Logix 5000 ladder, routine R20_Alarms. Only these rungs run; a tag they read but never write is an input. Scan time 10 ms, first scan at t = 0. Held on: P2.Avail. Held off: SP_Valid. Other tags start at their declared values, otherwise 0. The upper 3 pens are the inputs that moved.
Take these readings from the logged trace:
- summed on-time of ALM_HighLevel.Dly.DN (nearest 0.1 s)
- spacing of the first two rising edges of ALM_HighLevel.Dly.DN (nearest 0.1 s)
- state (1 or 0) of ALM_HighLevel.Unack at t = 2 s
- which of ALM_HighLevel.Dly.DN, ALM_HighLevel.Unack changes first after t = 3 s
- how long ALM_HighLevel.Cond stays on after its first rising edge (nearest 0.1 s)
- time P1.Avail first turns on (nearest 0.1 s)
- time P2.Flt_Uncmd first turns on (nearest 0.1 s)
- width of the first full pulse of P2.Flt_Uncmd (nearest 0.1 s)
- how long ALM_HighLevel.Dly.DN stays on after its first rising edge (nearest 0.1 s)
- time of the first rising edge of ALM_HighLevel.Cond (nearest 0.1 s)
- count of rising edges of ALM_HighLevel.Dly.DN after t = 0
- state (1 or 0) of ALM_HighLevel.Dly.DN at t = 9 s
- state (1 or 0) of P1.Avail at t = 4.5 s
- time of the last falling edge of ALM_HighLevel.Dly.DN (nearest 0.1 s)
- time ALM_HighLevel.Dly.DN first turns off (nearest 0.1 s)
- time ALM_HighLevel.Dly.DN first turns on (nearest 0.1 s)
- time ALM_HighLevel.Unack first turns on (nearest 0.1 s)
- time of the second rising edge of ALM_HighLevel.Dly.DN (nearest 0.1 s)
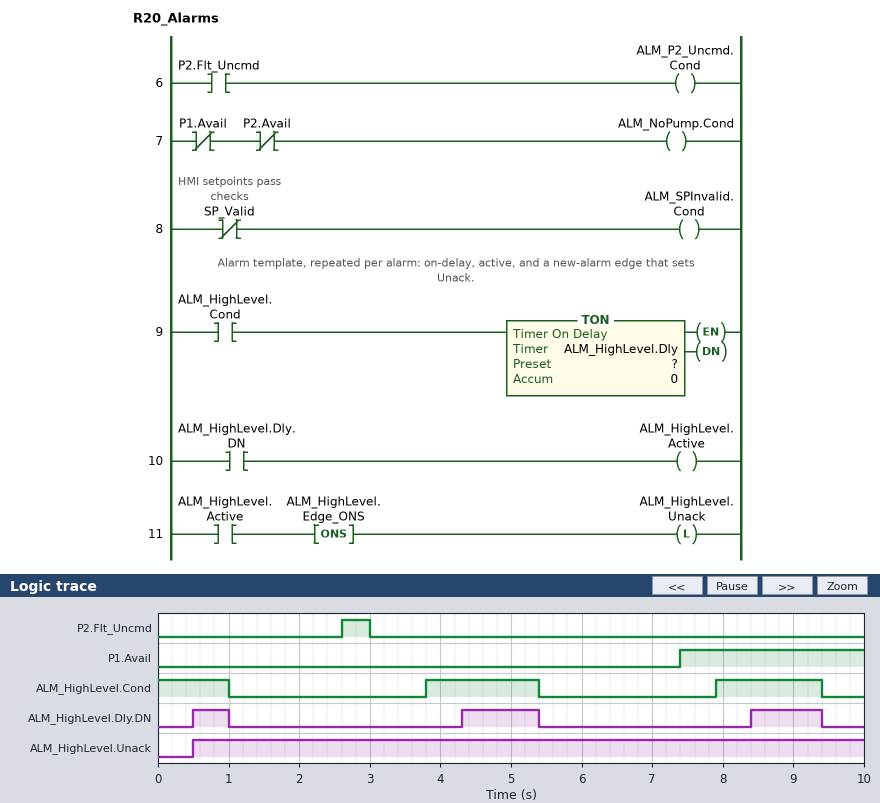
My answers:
2.6 s
3.8 s
1
ALM_HighLevel.Dly.DN
1.6 s
7.4 s
2.6 s
0.4 s
0.5 s
3.8 s
3
1
0
9.4 s
1.0 s
0.5 s
0.5 s
4.3 s
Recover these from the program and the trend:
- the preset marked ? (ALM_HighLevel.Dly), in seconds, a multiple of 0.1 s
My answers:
0.5 s
